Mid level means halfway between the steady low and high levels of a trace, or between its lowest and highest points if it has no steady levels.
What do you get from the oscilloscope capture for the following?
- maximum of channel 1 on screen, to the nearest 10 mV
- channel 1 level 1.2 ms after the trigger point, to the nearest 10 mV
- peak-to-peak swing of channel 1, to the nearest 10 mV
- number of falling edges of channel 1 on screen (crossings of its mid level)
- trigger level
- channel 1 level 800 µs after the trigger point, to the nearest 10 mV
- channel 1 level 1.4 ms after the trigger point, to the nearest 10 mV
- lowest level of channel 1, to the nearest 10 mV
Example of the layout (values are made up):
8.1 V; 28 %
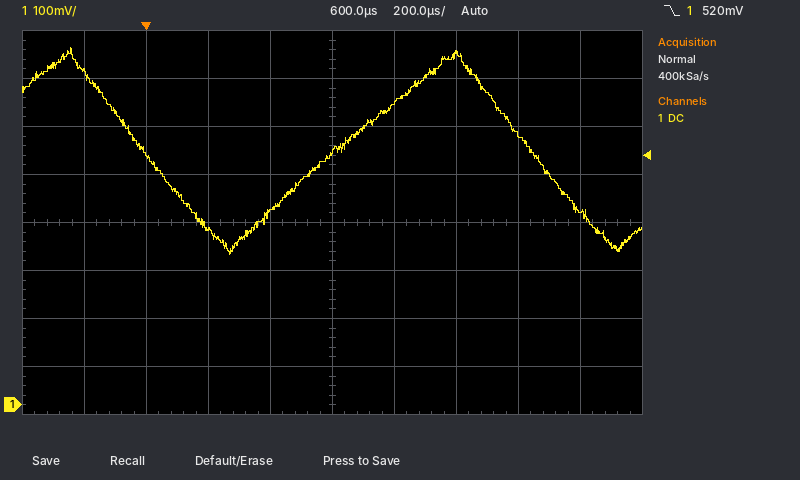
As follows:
740 mV; 560 mV; 430 mV; 2; 520 mV; 630 mV; 400 mV; 310 mV
